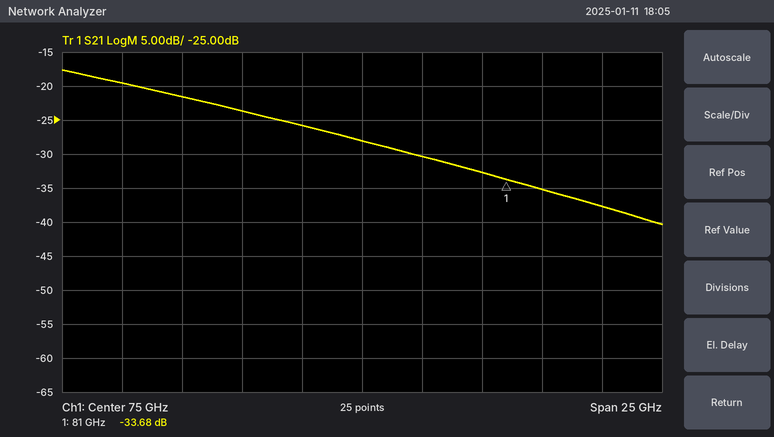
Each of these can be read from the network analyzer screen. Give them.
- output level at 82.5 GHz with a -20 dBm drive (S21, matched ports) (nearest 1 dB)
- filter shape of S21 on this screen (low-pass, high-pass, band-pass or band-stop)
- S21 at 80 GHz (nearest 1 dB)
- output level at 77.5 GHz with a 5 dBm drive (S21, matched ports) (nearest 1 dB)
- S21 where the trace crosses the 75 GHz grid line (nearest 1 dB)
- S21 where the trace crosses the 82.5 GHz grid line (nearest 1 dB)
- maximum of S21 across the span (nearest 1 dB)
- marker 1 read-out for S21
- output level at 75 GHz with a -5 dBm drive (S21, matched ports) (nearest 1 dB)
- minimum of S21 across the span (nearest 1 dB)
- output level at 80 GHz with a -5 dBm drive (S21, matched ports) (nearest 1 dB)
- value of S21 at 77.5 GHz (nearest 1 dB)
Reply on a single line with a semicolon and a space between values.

-55 dBm; low-pass; -33 dB; -25 dBm; -28 dB; -35 dB; -18 dB; -33.68 dB; -33 dBm; -40 dB; -38 dBm; -30 dB
